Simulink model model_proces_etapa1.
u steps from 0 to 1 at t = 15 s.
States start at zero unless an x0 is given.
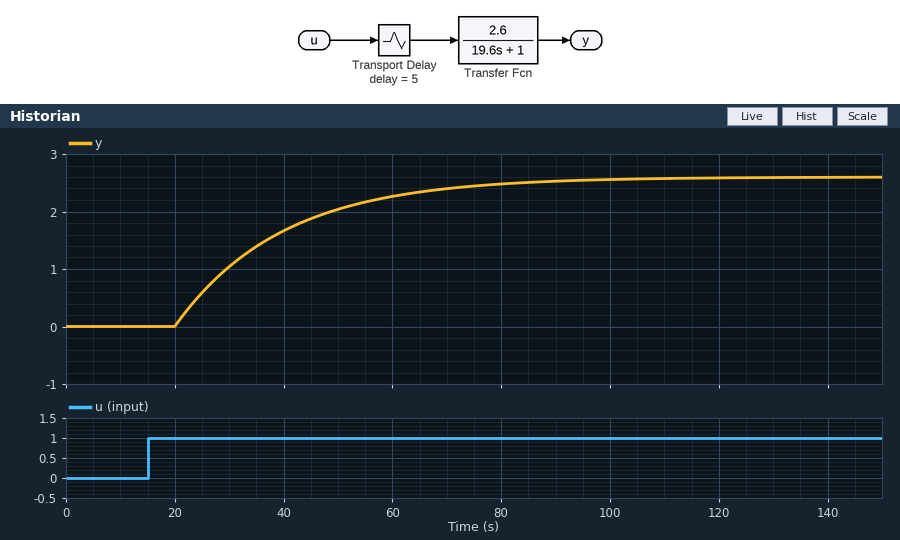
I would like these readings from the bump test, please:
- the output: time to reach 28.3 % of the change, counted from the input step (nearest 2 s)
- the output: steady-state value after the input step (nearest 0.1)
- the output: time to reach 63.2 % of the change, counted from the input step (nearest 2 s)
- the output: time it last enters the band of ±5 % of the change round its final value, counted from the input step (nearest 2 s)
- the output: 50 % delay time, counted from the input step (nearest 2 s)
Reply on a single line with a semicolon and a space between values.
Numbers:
12 s; 2.6; 24 s; 64 s; 18 s
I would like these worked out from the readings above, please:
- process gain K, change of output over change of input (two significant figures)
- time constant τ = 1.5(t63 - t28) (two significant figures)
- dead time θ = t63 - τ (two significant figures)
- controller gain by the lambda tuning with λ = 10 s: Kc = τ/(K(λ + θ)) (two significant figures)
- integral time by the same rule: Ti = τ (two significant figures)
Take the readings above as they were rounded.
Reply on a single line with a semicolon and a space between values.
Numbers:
2.6; 18 s; 6.0 s; 0.43; 18 s
